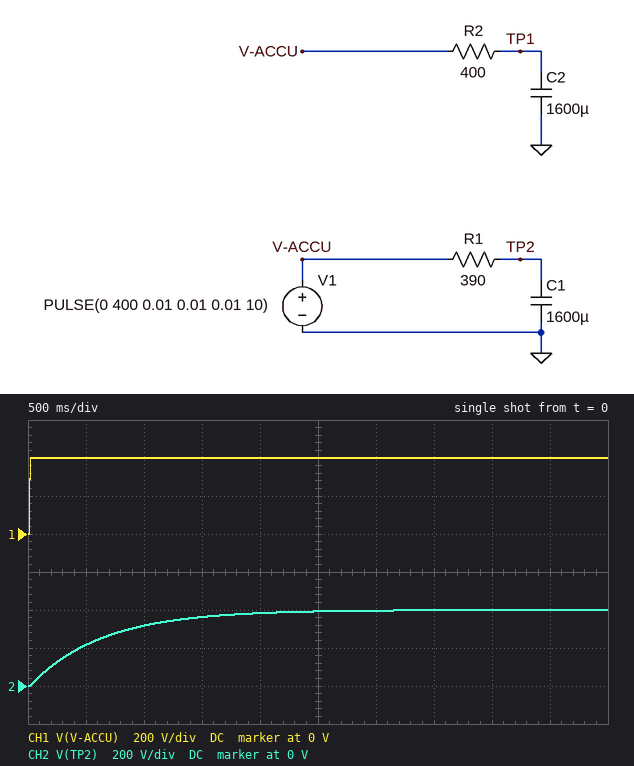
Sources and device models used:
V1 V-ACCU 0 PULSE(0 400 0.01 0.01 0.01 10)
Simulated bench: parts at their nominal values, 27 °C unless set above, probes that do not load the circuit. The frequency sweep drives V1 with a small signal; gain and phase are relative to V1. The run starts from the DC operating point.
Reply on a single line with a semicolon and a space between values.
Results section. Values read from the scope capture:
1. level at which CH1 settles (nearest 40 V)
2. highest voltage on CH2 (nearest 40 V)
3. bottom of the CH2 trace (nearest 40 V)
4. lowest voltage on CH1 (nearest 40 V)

400 V; 400 V; 0 V; 0 V
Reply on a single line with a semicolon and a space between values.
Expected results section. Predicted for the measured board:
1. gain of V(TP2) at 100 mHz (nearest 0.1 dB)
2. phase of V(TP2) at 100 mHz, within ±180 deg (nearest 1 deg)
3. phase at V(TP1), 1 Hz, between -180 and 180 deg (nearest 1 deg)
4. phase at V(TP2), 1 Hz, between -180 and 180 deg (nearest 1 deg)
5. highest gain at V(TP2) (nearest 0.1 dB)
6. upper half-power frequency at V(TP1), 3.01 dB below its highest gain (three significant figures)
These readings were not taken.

-0.6 dB; -21 deg; -76 deg; -76 deg; 0 dB; 249 mHz
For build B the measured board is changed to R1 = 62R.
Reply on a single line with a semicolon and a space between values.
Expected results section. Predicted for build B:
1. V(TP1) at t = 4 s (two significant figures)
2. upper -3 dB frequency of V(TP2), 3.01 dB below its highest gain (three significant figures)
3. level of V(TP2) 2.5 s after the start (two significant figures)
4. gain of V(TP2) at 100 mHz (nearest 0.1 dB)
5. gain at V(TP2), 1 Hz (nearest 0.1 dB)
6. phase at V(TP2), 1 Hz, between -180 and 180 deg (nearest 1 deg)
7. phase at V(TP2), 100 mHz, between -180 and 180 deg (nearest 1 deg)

400 V; 1.60 Hz; 400 V; 0 dB; -1.4 dB; -32 deg; -4 deg
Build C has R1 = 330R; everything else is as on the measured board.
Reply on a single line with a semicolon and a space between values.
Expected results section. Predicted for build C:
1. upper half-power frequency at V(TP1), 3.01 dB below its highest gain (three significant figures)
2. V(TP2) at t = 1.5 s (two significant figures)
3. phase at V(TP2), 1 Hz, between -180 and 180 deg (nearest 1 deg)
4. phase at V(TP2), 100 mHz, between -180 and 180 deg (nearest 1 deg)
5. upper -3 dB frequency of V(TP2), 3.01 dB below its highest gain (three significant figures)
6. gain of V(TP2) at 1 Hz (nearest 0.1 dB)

249 mHz; 380 V; -73 deg; -18 deg; 301 mHz; -10.8 dB
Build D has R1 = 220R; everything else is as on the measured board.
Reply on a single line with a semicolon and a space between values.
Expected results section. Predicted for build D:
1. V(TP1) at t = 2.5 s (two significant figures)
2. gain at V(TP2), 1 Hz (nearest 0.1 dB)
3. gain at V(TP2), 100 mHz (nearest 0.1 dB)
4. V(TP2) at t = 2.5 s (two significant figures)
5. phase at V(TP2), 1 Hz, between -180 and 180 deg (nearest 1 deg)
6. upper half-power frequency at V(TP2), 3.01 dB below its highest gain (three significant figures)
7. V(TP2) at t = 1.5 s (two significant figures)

390 V; -7.7 dB; -0.2 dB; 400 V; -66 deg; 452 mHz; 390 V
